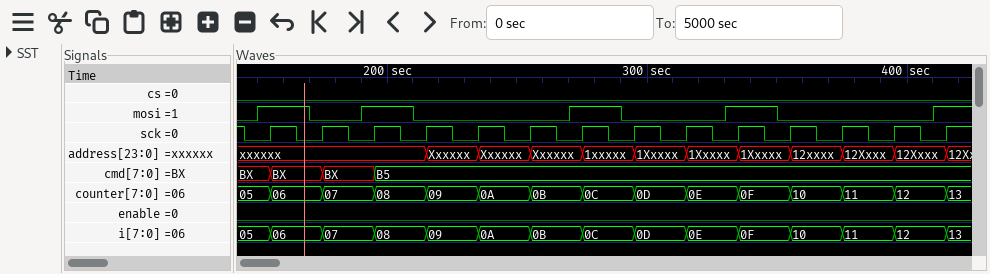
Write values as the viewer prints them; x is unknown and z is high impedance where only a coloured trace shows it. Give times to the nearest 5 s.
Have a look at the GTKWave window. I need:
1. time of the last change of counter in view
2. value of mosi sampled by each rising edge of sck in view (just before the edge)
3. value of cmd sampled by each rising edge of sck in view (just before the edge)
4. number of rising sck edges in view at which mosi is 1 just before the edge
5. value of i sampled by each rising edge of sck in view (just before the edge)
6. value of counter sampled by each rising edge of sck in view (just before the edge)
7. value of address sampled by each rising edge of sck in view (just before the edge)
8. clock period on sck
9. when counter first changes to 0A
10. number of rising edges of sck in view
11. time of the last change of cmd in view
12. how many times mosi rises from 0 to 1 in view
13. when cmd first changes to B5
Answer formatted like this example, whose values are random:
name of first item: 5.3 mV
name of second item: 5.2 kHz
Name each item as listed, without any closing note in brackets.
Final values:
time of the last change of counter in view: 415 s
value of mosi sampled by each rising edge of sck in view: 1 0 1 0 0 0 1 0 0 1 0 0 0 1
value of cmd sampled by each rising edge of sck in view: BX, BX, BX, B5, B5, B5, B5, B5, B5, B5, B5, B5, B5, B5
number of rising sck edges in view at which mosi is 1 just before the edge: 5
value of i sampled by each rising edge of sck in view: 05, 06, 07, 08, 09, 0A, 0B, 0C, 0D, 0E, 0F, 10, 11, 12
value of counter sampled by each rising edge of sck in view: 05, 06, 07, 08, 09, 0A, 0B, 0C, 0D, 0E, 0F, 10, 11, 12
value of address sampled by each rising edge of sck in view: xxxxxx, xxxxxx, xxxxxx, xxxxxx, Xxxxxx, Xxxxxx, Xxxxxx, 1xxxxx, 1Xxxxx, 1Xxxxx, 1Xxxxx, 12xxxx, 12Xxxx, 12Xxxx
clock period on sck: 20 s
when counter first changes to 0A: 235 s
number of rising edges of sck in view: 14
time of the last change of cmd in view: 195 s
how many times mosi rises from 0 to 1 in view: 5
when cmd first changes to B5: 195 s
